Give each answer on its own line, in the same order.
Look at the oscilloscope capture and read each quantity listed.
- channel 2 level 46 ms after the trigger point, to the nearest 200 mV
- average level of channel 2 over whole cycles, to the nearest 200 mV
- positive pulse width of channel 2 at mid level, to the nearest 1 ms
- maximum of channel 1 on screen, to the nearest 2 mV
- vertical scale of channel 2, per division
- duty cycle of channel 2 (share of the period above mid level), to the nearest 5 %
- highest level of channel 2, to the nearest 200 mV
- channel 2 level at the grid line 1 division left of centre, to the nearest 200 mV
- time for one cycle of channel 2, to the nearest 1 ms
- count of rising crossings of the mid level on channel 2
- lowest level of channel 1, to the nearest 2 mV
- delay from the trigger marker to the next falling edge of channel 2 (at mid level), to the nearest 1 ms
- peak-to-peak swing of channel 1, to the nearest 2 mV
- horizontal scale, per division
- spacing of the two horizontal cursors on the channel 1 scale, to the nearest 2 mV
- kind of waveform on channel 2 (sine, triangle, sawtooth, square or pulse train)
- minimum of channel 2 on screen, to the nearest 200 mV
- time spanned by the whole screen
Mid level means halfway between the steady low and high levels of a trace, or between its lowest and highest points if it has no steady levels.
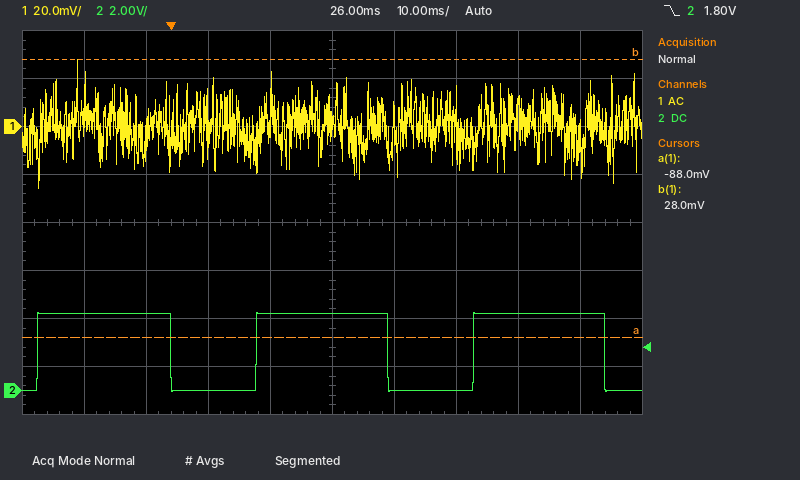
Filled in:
0.0 V
2.0 V
21 ms
28 mV
2 V
60 %
3.2 V
3.2 V
35 ms
3
-26 mV
35 ms
54 mV
10 ms
116 mV
pulse train
0.0 V
100 ms
